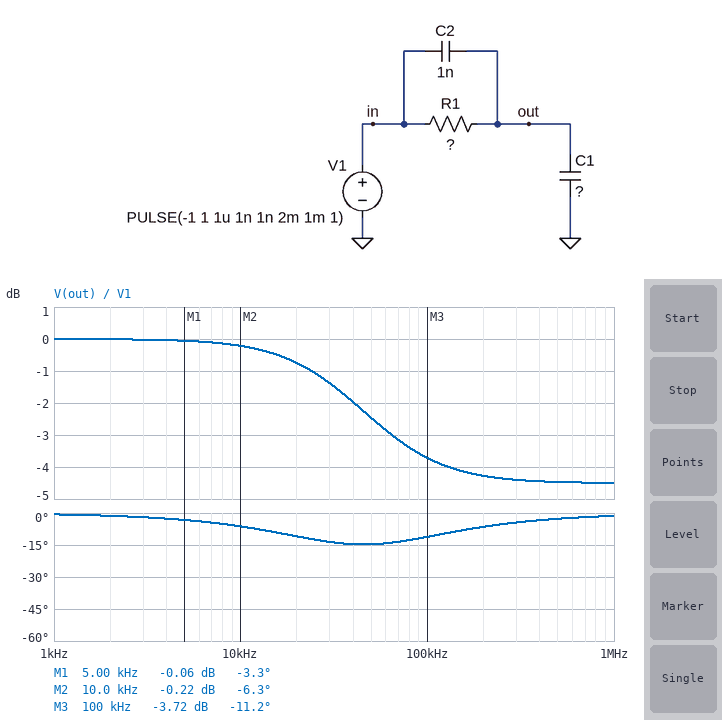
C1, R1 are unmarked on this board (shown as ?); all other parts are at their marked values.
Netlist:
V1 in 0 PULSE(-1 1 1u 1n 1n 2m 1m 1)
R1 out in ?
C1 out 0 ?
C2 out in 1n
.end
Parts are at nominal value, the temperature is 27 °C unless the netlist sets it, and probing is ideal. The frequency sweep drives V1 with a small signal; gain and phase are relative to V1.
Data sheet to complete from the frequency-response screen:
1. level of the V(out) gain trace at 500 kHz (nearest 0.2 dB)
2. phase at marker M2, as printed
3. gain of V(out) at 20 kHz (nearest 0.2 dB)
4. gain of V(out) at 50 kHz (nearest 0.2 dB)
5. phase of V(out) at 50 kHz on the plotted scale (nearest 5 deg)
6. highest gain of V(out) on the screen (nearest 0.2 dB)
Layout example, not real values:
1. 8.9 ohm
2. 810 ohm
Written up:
1. -4.4 dB
2. -6.3 deg
3. -0.8 dB
4. -2.4 dB
5. -15 deg
6. 0 dB
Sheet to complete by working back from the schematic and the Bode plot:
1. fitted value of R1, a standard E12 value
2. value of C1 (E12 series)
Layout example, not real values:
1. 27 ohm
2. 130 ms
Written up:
1. 2.7 kΩ
2. 680 pF
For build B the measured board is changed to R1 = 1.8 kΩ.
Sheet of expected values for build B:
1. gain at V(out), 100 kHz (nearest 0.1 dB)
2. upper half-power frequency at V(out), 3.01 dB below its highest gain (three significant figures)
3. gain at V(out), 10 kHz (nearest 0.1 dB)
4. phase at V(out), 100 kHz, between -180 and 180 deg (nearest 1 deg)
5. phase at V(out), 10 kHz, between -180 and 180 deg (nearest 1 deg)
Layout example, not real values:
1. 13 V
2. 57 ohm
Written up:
1. -3.1 dB
2. 97.5 kHz
3. -0.1 dB
4. -14 deg
5. -4 deg
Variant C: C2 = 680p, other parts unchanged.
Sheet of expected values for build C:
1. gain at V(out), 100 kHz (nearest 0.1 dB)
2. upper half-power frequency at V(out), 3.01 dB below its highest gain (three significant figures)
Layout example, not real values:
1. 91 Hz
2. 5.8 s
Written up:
1. -4.3 dB
2. 61.3 kHz
